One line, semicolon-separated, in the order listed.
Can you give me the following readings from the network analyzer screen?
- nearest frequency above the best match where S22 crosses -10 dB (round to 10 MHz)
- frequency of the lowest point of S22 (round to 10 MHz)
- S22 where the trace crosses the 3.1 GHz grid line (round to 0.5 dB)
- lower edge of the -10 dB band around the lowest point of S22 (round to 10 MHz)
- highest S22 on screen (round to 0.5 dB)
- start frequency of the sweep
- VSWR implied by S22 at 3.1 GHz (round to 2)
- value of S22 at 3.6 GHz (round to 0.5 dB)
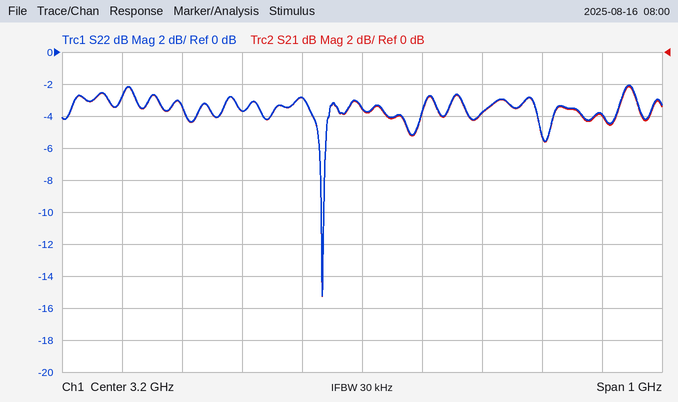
3.14 GHz; 3.13 GHz; -3.0 dB; 3.13 GHz; -2.0 dB; 2.7 GHz; 6; -4.0 dB
